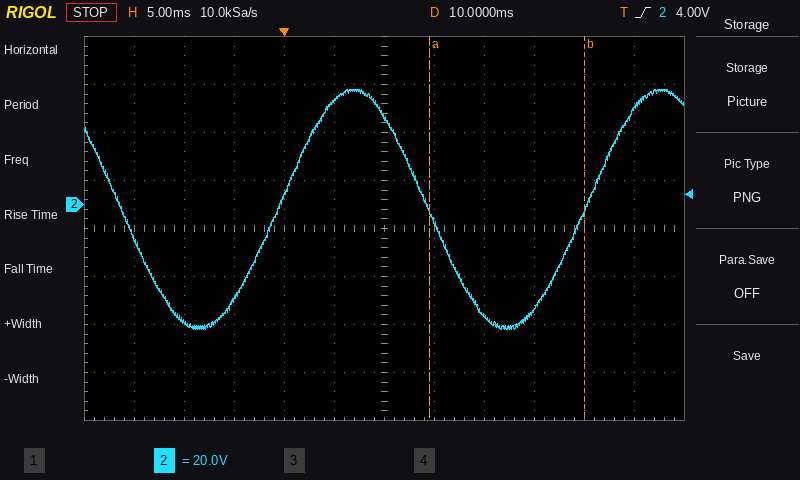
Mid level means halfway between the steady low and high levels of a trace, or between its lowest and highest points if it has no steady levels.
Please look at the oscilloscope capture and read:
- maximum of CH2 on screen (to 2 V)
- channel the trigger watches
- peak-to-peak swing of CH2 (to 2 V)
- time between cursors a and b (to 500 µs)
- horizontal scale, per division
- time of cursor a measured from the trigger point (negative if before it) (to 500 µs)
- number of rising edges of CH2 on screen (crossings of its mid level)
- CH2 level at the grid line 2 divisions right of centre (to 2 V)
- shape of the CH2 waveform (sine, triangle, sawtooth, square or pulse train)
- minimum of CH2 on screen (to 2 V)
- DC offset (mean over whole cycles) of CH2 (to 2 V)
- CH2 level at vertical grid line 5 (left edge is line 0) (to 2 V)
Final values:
48 V
CH2
100 V
15.5 ms
5 ms
+14.5 ms
2
-46 V
sine
-52 V
-2 V
44 V
